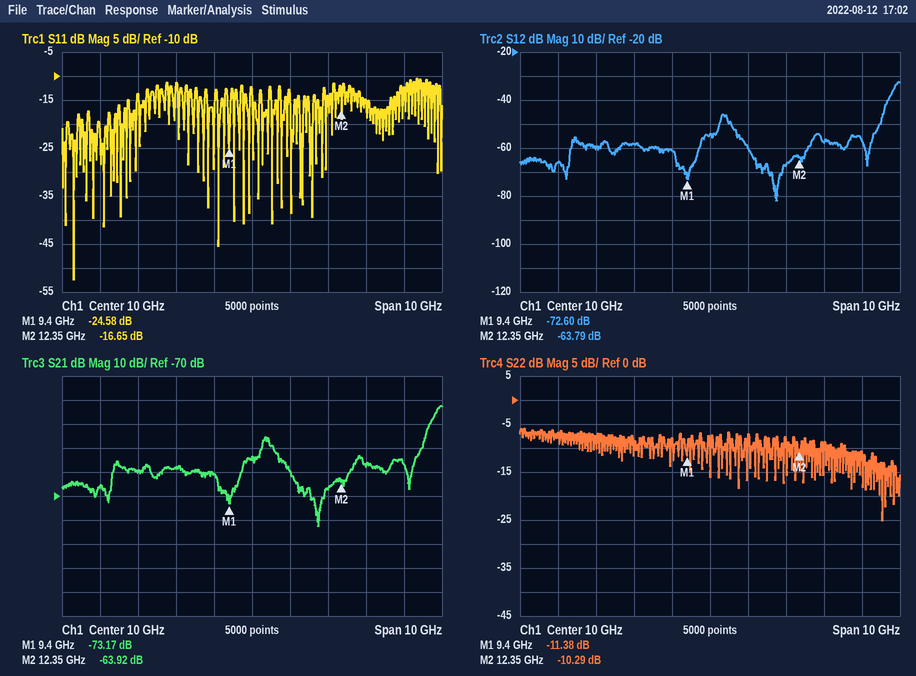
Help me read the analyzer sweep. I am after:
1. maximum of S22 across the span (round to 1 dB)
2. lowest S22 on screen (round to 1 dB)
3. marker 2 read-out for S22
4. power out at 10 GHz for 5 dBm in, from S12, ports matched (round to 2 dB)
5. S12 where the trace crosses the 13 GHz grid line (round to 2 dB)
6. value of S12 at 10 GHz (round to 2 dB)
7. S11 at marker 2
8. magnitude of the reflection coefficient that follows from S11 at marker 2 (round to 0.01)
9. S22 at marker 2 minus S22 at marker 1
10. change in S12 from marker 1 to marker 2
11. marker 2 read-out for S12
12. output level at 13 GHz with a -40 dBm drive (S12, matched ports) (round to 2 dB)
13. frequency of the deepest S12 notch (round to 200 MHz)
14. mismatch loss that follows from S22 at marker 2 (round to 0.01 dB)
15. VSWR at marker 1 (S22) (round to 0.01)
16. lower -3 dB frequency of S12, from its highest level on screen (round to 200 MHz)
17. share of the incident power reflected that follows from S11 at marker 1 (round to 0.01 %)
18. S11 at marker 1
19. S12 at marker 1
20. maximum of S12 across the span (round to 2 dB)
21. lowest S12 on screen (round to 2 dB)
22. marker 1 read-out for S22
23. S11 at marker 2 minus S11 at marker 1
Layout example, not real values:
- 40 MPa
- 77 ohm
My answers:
- -6 dB
- -25 dB
- -10.29 dB
- -50 dBm
- -58 dB
- -54 dB
- -16.65 dB
- 0.15
- 1.09 dB
- 8.81 dB
- -63.79 dB
- -98 dBm
- 11.8 GHz
- 0.43 dB
- 1.74
- 14.8 GHz
- 0.35 %
- -24.58 dB
- -72.60 dB
- -32 dB
- -82 dB
- -11.38 dB
- 7.93 dB
